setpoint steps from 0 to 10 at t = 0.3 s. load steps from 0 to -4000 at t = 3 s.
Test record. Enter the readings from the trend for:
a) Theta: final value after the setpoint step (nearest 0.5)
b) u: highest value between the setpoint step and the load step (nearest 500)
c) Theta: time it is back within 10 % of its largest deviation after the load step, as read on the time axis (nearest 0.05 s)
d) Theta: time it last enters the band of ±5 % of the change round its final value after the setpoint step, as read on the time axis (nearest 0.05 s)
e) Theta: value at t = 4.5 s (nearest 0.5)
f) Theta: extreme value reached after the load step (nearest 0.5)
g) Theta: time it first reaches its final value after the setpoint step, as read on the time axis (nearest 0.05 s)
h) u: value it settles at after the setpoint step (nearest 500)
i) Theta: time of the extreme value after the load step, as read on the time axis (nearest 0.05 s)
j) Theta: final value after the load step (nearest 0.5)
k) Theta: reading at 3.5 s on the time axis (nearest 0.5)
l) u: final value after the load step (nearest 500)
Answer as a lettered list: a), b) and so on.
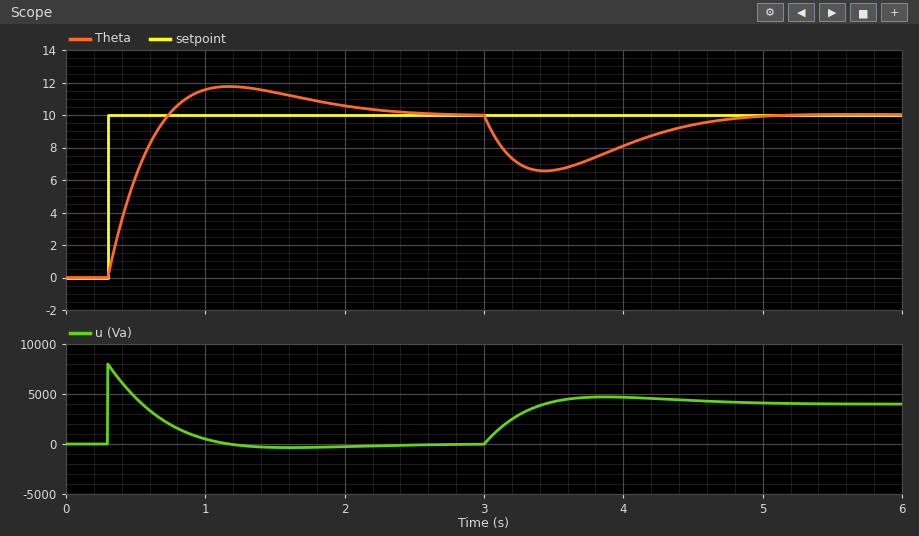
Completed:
a) 10.0
b) 8000
c) 4.70 s
d) 2.05 s
e) 9.5
f) 6.5
g) 0.75 s
h) 0
i) 3.45 s
j) 10.0
k) 6.5
l) 4000
